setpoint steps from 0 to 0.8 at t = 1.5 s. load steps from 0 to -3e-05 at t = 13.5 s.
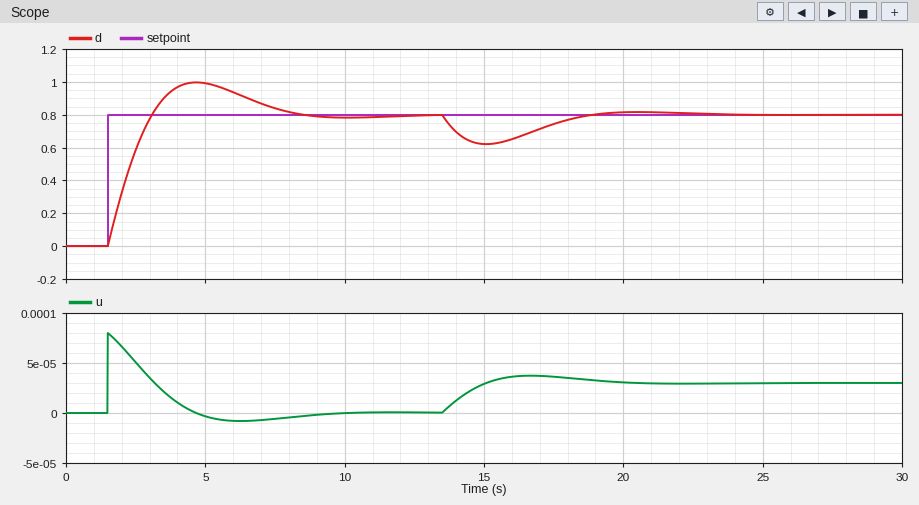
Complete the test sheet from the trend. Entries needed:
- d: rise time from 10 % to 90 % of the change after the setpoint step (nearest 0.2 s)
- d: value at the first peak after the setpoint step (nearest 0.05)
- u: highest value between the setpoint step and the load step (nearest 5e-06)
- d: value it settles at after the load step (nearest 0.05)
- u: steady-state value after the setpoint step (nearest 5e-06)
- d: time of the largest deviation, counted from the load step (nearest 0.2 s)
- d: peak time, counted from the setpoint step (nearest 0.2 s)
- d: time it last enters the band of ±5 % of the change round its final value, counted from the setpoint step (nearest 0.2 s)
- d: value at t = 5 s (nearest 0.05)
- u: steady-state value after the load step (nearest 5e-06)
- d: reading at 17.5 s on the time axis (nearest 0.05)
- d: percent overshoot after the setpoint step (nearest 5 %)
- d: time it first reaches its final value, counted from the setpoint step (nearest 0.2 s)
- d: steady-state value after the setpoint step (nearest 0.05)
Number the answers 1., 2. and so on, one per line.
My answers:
1. 1.2 s
2. 1.00
3. 0.000080
4. 0.80
5. 0.000000
6. 1.6 s
7. 3.2 s
8. 6.0 s
9. 1.00
10. 0.000030
11. 0.75
12. 25 %
13. 1.6 s
14. 0.80
